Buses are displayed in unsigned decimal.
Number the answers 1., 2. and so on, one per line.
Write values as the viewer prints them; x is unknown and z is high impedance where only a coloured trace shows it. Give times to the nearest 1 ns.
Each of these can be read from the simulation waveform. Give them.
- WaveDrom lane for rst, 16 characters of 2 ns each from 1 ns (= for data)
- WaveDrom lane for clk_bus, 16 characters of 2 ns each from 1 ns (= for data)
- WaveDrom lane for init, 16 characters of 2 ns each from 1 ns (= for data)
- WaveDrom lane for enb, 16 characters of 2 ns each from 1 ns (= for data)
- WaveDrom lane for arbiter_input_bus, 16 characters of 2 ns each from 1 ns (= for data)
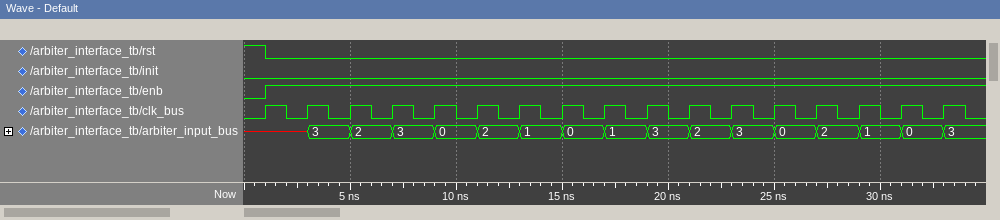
1. {name: 'rst', wave: '0...............'}
2. {name: 'clk_bus', wave: 'p...............'}
3. {name: 'init', wave: '0...............'}
4. {name: 'enb', wave: '1...............'}
5. {name: 'arbiter_input_bus', wave: 'x===============', data: '3 2 3 0 2 1 0 1 3 2 3 0 2 1 0'}
